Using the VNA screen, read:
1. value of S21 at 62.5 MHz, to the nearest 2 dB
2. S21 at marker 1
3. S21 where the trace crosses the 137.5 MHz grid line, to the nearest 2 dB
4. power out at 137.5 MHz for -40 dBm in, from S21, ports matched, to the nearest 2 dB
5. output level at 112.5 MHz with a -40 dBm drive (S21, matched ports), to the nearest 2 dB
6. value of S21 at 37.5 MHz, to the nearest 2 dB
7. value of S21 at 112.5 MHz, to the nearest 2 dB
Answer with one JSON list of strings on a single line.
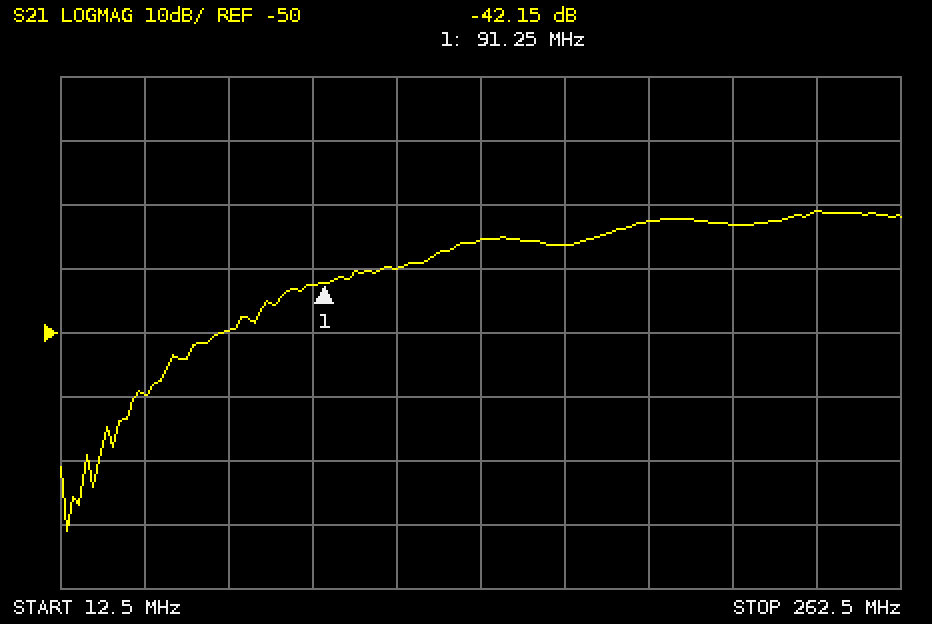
["-50 dB", "-42.15 dB", "-36 dB", "-76 dBm", "-80 dBm", "-60 dB", "-40 dB"]
